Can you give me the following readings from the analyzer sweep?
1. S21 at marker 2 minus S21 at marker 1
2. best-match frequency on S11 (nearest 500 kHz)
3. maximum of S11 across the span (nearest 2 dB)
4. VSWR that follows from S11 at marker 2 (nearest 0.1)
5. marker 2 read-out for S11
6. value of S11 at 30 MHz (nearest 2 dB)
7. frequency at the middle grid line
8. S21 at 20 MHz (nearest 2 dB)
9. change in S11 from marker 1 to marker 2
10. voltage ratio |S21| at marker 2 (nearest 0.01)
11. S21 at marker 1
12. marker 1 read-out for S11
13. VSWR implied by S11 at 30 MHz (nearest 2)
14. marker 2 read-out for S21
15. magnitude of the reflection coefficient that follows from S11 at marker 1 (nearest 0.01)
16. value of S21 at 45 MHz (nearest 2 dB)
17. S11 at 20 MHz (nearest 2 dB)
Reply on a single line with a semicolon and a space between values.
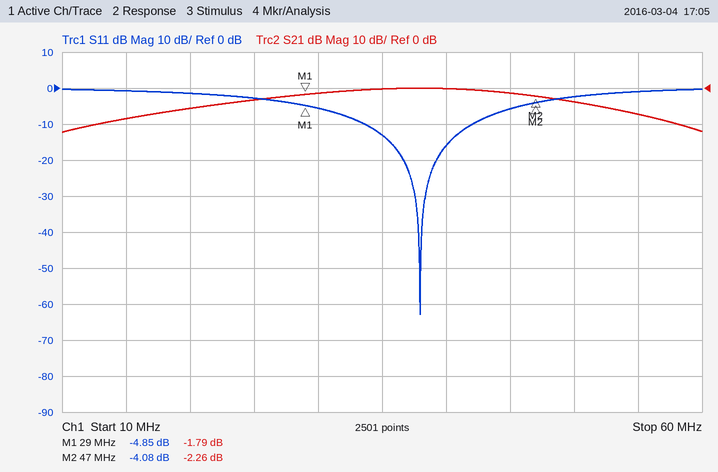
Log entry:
-0.47 dB; 38.0 MHz; 0 dB; 4.3; -4.08 dB; -6 dB; 35 MHz; -6 dB; 0.77 dB; 0.77; -1.79 dB; -4.85 dB; 4; -2.26 dB; 0.57; -2 dB; -2 dB
